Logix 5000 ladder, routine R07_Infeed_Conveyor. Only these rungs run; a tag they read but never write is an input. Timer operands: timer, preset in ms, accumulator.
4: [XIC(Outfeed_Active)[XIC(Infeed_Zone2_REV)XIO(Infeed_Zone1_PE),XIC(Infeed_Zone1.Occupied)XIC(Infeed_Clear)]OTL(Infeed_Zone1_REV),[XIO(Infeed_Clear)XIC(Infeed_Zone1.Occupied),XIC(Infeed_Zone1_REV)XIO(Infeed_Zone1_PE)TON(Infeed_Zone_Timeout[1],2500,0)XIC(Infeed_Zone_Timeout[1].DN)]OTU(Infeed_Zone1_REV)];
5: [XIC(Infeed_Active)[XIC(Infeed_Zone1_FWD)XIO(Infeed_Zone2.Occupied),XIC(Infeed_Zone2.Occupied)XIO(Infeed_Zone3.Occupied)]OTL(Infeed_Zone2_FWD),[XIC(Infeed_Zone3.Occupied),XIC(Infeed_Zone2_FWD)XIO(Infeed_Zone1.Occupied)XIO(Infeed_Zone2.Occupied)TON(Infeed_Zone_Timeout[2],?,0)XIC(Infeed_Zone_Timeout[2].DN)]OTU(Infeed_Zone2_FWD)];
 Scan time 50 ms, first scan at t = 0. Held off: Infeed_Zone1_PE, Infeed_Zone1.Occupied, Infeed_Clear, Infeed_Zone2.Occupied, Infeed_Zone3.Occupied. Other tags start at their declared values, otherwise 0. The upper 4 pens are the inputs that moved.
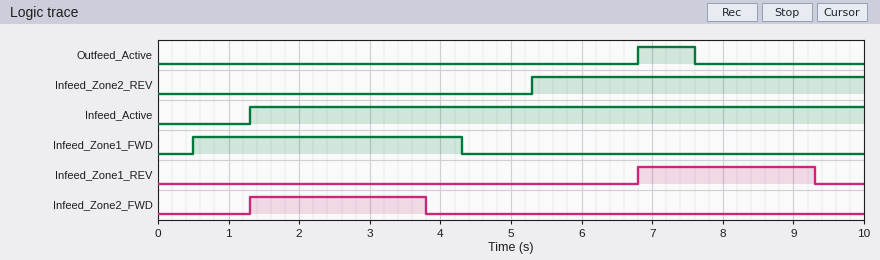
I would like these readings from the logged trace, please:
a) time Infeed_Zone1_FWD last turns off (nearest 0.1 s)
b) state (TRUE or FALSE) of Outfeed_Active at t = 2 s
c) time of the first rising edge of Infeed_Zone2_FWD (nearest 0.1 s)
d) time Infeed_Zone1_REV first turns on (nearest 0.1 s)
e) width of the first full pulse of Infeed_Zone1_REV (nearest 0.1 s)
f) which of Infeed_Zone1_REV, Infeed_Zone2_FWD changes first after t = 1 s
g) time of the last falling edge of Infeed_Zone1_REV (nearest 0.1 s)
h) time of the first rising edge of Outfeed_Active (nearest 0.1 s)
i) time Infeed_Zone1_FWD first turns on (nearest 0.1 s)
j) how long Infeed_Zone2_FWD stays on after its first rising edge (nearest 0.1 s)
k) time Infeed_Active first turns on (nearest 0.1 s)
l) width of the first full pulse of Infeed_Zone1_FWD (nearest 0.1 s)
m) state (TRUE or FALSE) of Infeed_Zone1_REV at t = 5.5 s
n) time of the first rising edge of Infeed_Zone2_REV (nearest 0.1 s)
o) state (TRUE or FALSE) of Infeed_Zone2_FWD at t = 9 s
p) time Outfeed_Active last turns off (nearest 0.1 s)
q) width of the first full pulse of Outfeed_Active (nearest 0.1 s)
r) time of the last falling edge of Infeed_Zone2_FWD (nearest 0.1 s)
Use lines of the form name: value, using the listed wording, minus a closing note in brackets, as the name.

time Infeed_Zone1_FWD last turns off: 4.3 s
state (TRUE or FALSE) of Outfeed_Active at t = 2 s: FALSE
time of the first rising edge of Infeed_Zone2_FWD: 1.3 s
time Infeed_Zone1_REV first turns on: 6.8 s
width of the first full pulse of Infeed_Zone1_REV: 2.5 s
which of Infeed_Zone1_REV, Infeed_Zone2_FWD changes first after t = 1 s: Infeed_Zone2_FWD
time of the last falling edge of Infeed_Zone1_REV: 9.3 s
time of the first rising edge of Outfeed_Active: 6.8 s
time Infeed_Zone1_FWD first turns on: 0.5 s
how long Infeed_Zone2_FWD stays on after its first rising edge: 2.5 s
time Infeed_Active first turns on: 1.3 s
width of the first full pulse of Infeed_Zone1_FWD: 3.8 s
state (TRUE or FALSE) of Infeed_Zone1_REV at t = 5.5 s: FALSE
time of the first rising edge of Infeed_Zone2_REV: 5.3 s
state (TRUE or FALSE) of Infeed_Zone2_FWD at t = 9 s: FALSE
time Outfeed_Active last turns off: 7.6 s
width of the first full pulse of Outfeed_Active: 0.8 s
time of the last falling edge of Infeed_Zone2_FWD: 3.8 s
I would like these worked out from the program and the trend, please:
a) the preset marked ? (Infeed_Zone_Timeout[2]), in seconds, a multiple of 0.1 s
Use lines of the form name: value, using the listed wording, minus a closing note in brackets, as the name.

the preset marked ? (Infeed_Zone_Timeout[2]), in seconds, a multiple of 0.1 s: 2.5 s
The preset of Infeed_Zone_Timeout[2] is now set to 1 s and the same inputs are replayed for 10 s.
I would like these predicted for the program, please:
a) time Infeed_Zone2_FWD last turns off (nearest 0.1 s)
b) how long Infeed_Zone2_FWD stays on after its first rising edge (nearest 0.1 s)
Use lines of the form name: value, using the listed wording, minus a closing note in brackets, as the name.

time Infeed_Zone2_FWD last turns off: 2.3 s
how long Infeed_Zone2_FWD stays on after its first rising edge: 1.0 s
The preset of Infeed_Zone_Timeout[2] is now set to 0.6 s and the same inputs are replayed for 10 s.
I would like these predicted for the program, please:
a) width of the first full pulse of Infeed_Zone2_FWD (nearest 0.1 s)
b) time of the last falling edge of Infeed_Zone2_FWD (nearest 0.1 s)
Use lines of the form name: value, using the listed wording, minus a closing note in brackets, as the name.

width of the first full pulse of Infeed_Zone2_FWD: 0.6 s
time of the last falling edge of Infeed_Zone2_FWD: 1.9 s
